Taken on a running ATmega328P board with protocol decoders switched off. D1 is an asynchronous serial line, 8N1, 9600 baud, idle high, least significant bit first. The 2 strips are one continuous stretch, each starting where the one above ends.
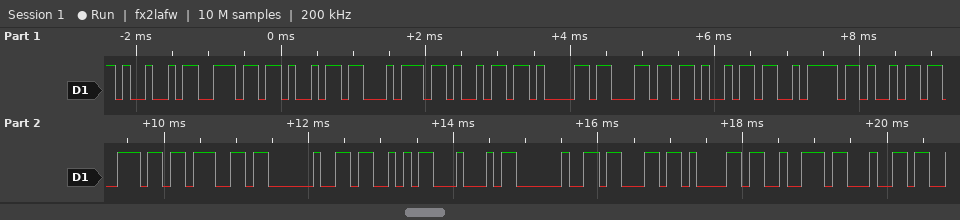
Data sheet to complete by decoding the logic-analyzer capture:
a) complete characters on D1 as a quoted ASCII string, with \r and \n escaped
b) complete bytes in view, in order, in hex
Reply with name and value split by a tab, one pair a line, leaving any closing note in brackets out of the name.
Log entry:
complete characters on D1 as a quoted ASCII string, with \r and \n escaped	"Initializing SD card"
complete bytes in view, in order, in hex	49 6E 69 74 69 61 6C 69 7A 69 6E 67 20 53 44 20 63 61 72 64
